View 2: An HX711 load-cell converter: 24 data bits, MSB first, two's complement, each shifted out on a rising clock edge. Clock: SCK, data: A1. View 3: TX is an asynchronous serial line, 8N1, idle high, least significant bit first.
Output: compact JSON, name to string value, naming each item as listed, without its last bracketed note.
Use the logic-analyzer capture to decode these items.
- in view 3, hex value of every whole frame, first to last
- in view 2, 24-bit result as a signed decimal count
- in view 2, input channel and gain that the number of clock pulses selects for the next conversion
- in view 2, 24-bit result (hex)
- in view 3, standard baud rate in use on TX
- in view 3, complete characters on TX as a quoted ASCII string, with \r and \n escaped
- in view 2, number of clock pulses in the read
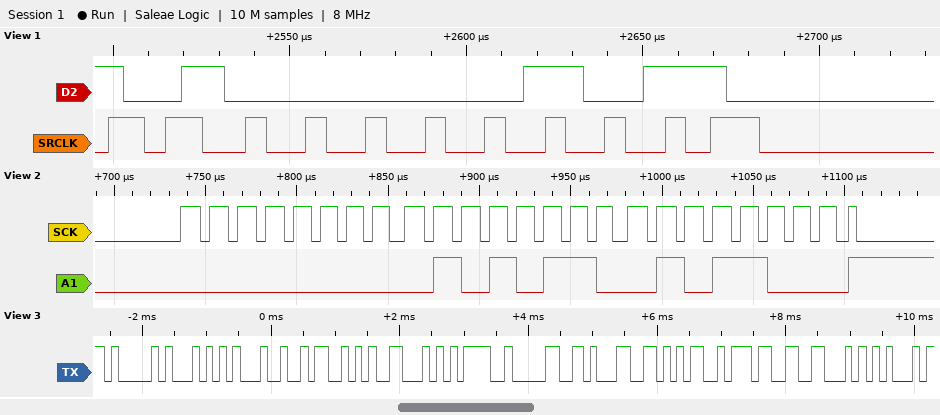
{"in view 3, hex value of every whole frame, first to last": "41 54 24 53 46 3D 30 31 35 37 46 45", "in view 2, 24-bit result as a signed decimal count": "22104", "in view 2, input channel and gain that the number of clock pulses selects for the next conversion": "channel A, gain 128", "in view 2, 24-bit result": "0x005658", "in view 3, standard baud rate in use on TX": "9600 baud", "in view 3, complete characters on TX as a quoted ASCII string, with \\r and \\n escaped": "\"AT$SF=0157FE\"", "in view 2, number of clock pulses in the read": "25"}
